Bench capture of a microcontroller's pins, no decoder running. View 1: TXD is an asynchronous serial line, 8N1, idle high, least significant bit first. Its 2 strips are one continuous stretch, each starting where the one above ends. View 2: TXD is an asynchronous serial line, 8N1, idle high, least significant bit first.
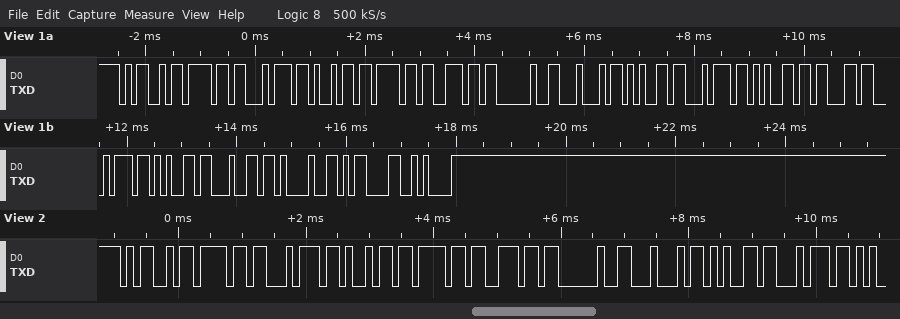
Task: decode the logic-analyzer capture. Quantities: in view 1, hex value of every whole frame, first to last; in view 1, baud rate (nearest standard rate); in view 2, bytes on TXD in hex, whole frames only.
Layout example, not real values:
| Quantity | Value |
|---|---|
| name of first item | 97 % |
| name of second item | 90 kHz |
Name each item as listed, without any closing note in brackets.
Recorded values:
| Quantity | Value |
|---|---|
| in view 1, hex value of every whole frame, first to last | 0x4D 0x6F 0x74 0x69 0x6F 0x6E 0x20 0x44 0x65 0x74 0x65 0x63 0x74 0x65 0x64 0x21 0x0D 0x0A |
| in view 1, baud rate | 9600 baud |
| in view 2, bytes on TXD in hex, whole frames only | 4D 6F 74 69 6F 6E 20 44 65 74 |
